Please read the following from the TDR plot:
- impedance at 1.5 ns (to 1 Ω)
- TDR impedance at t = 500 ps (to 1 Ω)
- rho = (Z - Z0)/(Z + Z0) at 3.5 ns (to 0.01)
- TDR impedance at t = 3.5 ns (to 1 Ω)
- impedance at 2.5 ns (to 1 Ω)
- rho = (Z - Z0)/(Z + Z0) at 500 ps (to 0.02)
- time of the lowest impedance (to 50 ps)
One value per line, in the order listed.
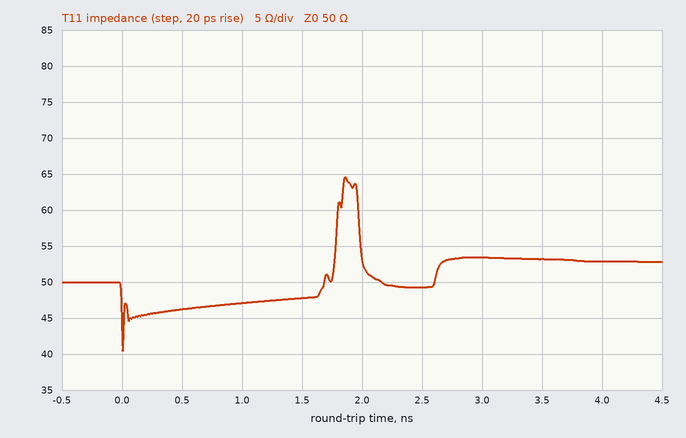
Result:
48 Ω
46 Ω
+0.03
53 Ω
49 Ω
-0.04
0 ps
